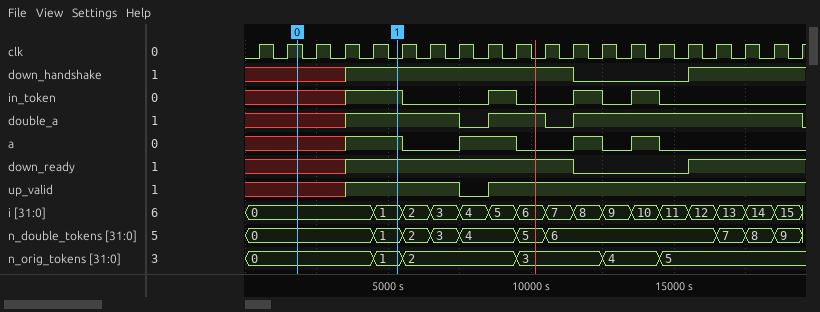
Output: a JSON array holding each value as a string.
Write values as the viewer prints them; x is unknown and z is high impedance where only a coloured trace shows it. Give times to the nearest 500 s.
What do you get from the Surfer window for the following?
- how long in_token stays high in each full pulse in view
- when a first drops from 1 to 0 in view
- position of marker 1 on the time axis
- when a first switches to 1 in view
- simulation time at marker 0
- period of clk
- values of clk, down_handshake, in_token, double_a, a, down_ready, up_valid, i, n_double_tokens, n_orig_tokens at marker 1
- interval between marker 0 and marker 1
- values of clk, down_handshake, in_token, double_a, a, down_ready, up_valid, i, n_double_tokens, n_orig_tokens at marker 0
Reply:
["1000 s, 1000 s, 1000 s", "5500 s", "5500 s", "3500 s", "2000 s", "1000 s", "clk=0, down_handshake=1, in_token=1, double_a=1, a=1, down_ready=1, up_valid=1, i=1, n_double_tokens=1, n_orig_tokens=1", "3500 s", "clk=1, down_handshake=x, in_token=x, double_a=x, a=x, down_ready=x, up_valid=x, i=0, n_double_tokens=0, n_orig_tokens=0"]
